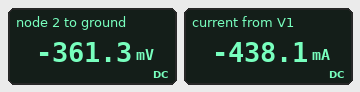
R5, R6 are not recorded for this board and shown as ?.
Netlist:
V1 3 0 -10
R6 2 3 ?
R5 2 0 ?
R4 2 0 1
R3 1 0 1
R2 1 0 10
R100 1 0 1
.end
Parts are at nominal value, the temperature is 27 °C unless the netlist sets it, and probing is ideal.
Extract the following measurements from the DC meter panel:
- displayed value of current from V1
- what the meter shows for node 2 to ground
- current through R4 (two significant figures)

-438.1 mA
-361.3 mV
360 mA
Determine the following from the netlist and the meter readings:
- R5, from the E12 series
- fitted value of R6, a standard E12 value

4.7 Ω
22 Ω
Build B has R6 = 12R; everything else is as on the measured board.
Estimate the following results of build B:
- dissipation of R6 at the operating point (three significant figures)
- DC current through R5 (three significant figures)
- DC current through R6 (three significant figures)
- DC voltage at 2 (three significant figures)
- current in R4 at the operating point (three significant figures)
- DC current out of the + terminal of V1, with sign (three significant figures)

7.30 W
137 mA
780 mA
-643 mV
643 mA
-780 mA
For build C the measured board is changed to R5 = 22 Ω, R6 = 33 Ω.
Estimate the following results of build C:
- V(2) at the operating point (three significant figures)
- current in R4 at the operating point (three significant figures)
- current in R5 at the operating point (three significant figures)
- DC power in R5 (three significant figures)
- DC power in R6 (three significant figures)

-282 mV
282 mA
12.8 mA
3.61 mW
2.86 W
